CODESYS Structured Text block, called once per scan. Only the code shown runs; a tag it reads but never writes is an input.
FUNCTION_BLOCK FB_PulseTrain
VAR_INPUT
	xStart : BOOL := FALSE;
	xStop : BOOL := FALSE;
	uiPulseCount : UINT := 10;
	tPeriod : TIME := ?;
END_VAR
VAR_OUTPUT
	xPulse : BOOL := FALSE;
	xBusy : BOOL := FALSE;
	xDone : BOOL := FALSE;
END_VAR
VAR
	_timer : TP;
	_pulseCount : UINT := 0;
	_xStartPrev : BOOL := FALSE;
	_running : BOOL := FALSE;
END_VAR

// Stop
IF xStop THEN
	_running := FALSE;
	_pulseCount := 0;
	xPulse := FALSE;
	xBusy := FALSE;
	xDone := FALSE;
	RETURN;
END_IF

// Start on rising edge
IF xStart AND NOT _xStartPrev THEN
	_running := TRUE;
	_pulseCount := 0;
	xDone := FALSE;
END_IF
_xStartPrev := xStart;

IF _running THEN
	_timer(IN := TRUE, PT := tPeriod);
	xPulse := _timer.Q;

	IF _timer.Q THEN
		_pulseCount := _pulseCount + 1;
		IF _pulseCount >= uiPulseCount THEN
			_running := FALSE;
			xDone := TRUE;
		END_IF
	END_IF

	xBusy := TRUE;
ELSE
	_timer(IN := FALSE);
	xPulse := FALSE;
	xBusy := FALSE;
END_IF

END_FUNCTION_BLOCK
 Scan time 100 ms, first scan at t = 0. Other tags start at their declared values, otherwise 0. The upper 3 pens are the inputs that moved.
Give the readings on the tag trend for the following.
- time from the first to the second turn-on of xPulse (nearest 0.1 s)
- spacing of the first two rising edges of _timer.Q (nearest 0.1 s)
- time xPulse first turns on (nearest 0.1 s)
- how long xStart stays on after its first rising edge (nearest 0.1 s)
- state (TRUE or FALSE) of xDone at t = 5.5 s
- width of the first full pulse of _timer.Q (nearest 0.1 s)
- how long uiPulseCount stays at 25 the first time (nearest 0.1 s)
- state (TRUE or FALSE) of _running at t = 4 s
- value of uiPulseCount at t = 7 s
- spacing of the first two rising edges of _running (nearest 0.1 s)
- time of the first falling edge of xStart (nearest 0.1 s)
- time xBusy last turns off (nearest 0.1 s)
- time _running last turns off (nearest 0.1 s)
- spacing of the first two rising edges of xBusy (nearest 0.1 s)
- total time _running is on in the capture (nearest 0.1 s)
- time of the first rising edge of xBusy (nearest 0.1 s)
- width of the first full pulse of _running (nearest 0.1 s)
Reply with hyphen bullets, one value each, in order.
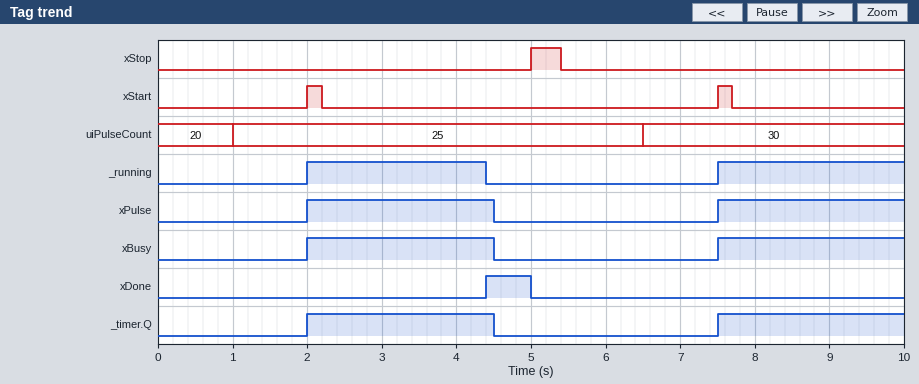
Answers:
- 5.5 s
- 5.5 s
- 2.0 s
- 0.2 s
- FALSE
- 2.5 s
- 5.5 s
- TRUE
- 30
- 5.5 s
- 2.2 s
- 4.5 s
- 4.4 s
- 5.5 s
- 4.9 s
- 2.0 s
- 2.4 s
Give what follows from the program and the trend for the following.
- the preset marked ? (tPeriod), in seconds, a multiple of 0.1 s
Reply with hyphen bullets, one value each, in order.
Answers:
- 2.5 s
